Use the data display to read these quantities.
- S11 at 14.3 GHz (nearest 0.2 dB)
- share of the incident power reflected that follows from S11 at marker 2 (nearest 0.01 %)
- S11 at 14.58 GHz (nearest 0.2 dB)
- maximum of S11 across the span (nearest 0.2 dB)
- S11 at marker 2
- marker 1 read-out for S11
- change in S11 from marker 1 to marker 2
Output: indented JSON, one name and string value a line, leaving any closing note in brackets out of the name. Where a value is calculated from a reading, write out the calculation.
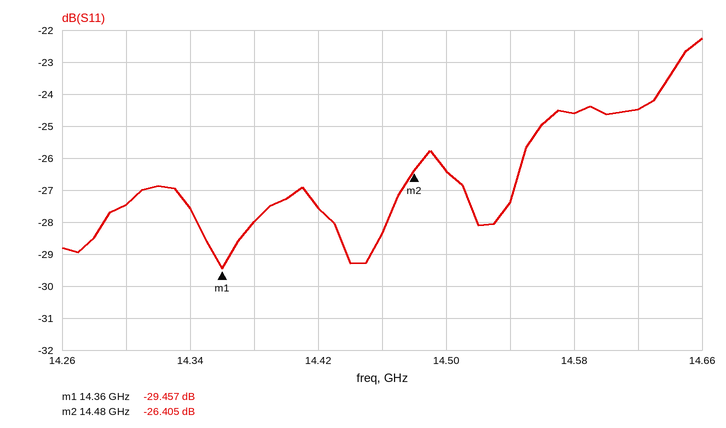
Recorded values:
{
  "S11 at 14.3 GHz": "-27.4 dB",
  "share of the incident power reflected that follows from S11 at marker 2": "10^(-26.405/10) ≈ 0.23 %",
  "S11 at 14.58 GHz": "-24.6 dB",
  "maximum of S11 across the span": "-22.2 dB",
  "S11 at marker 2": "-26.405 dB",
  "marker 1 read-out for S11": "-29.457 dB",
  "change in S11 from marker 1 to marker 2": "-26.405 − (-29.457) = 3.052 dB"
}
